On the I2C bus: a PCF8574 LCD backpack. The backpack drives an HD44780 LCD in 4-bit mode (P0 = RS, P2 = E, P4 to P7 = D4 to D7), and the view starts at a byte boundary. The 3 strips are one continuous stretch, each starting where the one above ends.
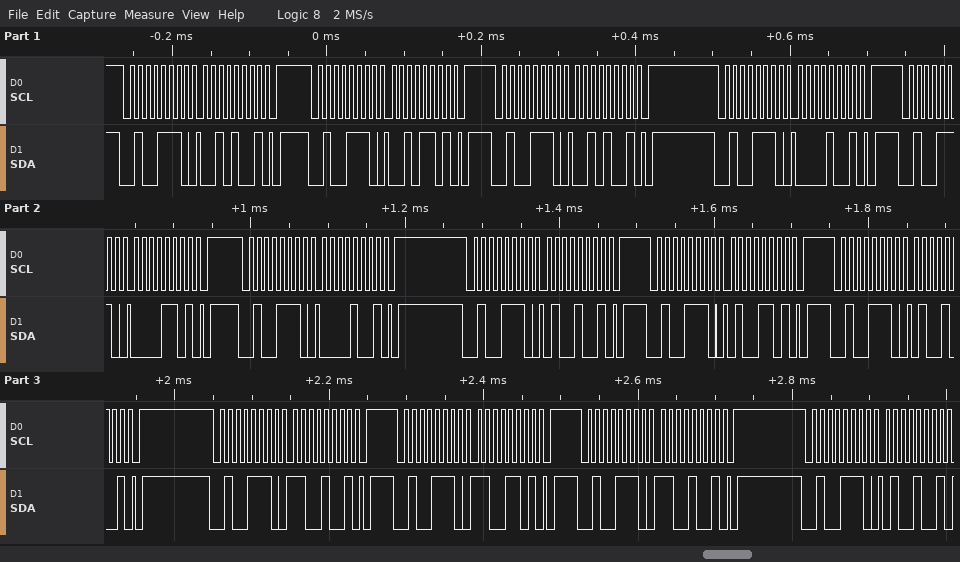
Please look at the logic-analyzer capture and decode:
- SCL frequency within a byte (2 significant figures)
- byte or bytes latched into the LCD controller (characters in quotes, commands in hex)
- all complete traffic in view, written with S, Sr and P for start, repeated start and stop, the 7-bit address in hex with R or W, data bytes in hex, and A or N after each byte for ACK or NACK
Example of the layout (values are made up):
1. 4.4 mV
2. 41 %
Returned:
1. 100 kHz
2. ' ' 'L'
3. S 27W A 29 A P S 27W A 2D A P S 27W A 29 A P S 27W A 09 A P S 27W A 0D A P S 27W A 09 A P S 27W A 49 A P S 27W A 4D A P S 27W A 49 A P S 27W A C9 A P S 27W A CD A P S 27W A C9 A P S 27W A 49 A
